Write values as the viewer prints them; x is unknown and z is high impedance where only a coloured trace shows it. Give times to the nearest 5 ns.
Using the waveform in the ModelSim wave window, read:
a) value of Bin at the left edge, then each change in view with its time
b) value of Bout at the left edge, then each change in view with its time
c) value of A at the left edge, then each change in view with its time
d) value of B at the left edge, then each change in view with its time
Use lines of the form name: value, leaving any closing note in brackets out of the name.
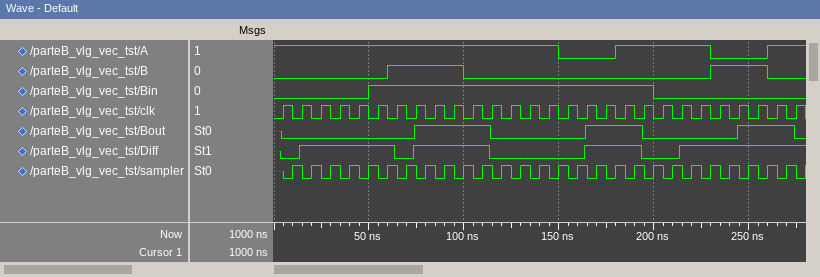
value of Bin at the left edge, then each change in view with its time: 0, 1 at 50 ns, 0 at 200 ns
value of Bout at the left edge, then each change in view with its time: x, 0 at 5 ns, 1 at 75 ns, 0 at 115 ns, 1 at 165 ns, 0 at 195 ns, 1 at 245 ns, 0 at 275 ns
value of A at the left edge, then each change in view with its time: 1, 0 at 150 ns, 1 at 180 ns, 0 at 230 ns, 1 at 260 ns
value of B at the left edge, then each change in view with its time: 0, 1 at 60 ns, 0 at 100 ns, 1 at 230 ns, 0 at 260 ns
